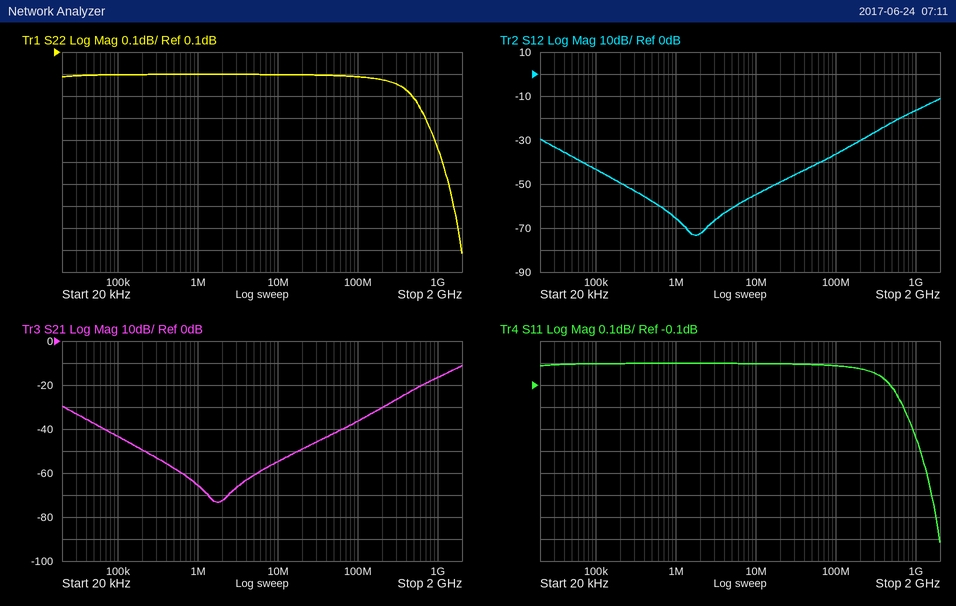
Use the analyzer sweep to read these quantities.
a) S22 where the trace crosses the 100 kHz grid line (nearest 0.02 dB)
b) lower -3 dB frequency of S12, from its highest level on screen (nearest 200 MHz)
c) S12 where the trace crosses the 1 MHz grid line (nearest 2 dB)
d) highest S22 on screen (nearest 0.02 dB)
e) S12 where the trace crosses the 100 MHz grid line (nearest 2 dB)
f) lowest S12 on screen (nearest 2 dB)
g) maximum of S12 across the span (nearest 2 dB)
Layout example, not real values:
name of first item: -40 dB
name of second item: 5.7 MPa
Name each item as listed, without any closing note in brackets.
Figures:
S22 where the trace crosses the 100 kHz grid line: 0.00 dB
lower -3 dB frequency of S12, from its highest level on screen: 1.4 GHz
S12 where the trace crosses the 1 MHz grid line: -66 dB
highest S22 on screen: 0.00 dB
S12 where the trace crosses the 100 MHz grid line: -36 dB
lowest S12 on screen: -74 dB
maximum of S12 across the span: -12 dB
